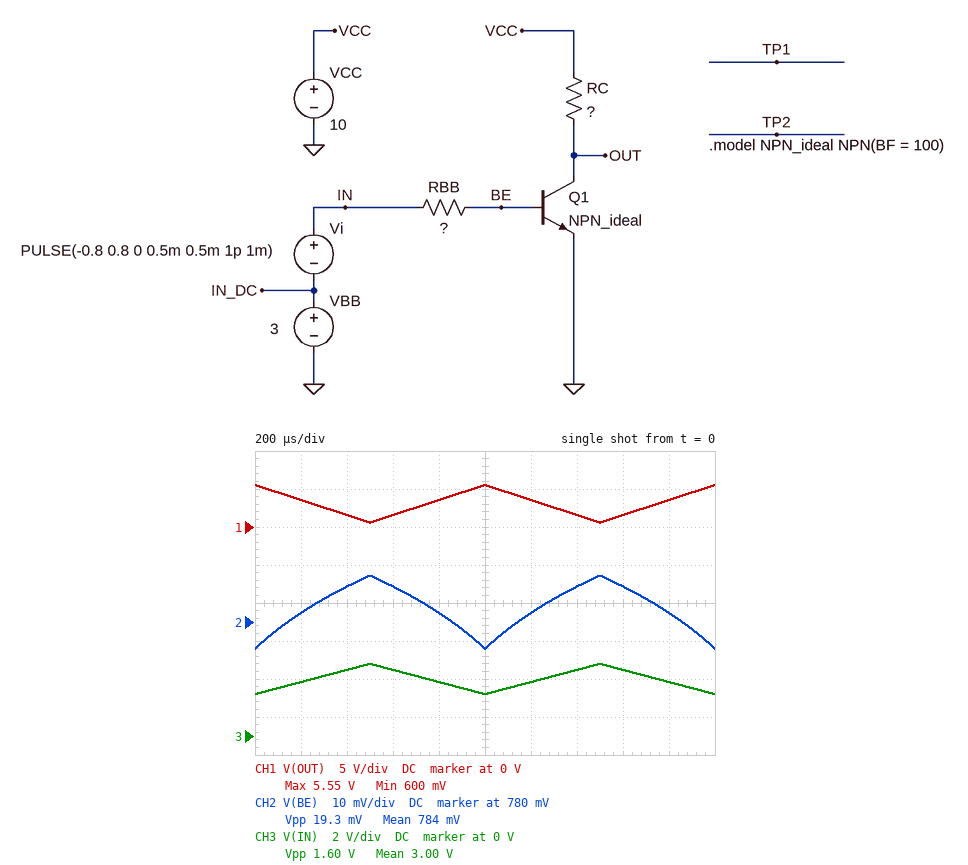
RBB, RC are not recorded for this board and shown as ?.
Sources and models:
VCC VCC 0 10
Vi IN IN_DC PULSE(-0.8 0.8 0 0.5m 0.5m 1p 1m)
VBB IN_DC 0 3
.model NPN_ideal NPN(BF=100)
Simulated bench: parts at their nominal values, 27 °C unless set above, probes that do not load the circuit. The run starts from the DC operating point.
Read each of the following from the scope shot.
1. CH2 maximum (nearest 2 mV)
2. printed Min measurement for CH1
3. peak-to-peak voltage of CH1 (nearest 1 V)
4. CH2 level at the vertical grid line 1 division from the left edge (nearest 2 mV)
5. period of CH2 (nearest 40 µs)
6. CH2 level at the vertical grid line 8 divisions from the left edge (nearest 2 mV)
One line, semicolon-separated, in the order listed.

792 mV; 600 mV; 5 V; 782 mV; 1.00 ms; 790 mV
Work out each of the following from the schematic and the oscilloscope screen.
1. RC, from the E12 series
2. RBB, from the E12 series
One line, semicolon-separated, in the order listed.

4.7 kΩ; 150 kΩ
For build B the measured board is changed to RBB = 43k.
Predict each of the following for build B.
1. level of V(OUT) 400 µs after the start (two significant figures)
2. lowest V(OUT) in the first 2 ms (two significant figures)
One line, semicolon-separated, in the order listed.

100 mV; 99 mV
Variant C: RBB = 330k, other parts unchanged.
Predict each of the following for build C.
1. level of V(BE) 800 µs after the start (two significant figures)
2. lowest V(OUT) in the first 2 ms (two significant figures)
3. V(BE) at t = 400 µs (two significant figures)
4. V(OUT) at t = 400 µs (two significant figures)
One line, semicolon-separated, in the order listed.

760 mV; 5.7 V; 770 mV; 6.1 V
